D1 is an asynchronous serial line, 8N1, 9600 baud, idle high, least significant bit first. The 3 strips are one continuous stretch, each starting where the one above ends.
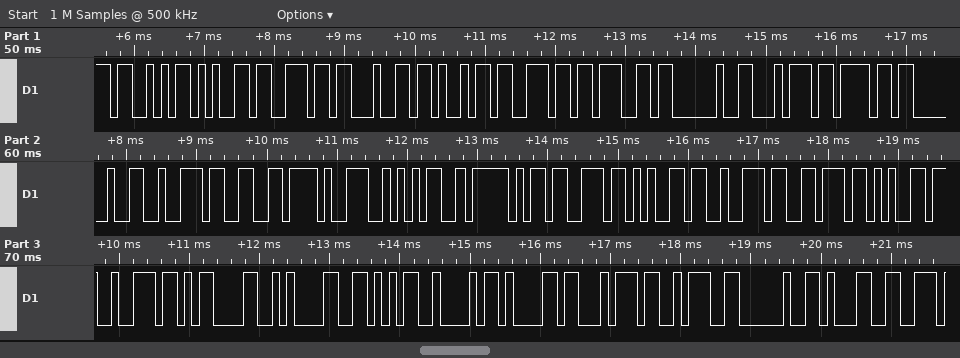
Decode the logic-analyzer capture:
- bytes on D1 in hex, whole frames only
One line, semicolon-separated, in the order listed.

53 65 6E 64 69 6E 67 20 74 6F 20 72 66 39 35 5F 73 65 72 76 65 72 0D 0A 56 42 61 74 3A 20 31
